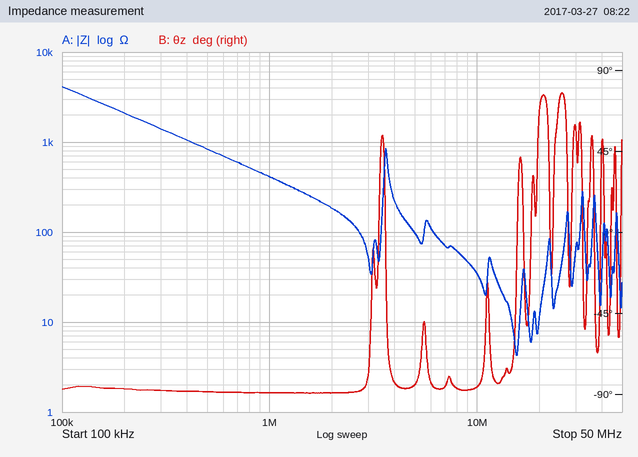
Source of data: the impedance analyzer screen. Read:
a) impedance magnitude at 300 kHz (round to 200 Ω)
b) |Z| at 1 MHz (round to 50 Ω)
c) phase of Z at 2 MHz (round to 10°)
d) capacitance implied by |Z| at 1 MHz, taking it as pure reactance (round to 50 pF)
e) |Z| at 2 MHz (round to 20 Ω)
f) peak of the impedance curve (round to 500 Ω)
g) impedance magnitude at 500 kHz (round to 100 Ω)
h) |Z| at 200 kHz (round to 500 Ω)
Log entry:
1.4 kΩ
400 Ω
-90°
400 pF
180 Ω
4.0 kΩ
800 Ω
2.0 kΩ
